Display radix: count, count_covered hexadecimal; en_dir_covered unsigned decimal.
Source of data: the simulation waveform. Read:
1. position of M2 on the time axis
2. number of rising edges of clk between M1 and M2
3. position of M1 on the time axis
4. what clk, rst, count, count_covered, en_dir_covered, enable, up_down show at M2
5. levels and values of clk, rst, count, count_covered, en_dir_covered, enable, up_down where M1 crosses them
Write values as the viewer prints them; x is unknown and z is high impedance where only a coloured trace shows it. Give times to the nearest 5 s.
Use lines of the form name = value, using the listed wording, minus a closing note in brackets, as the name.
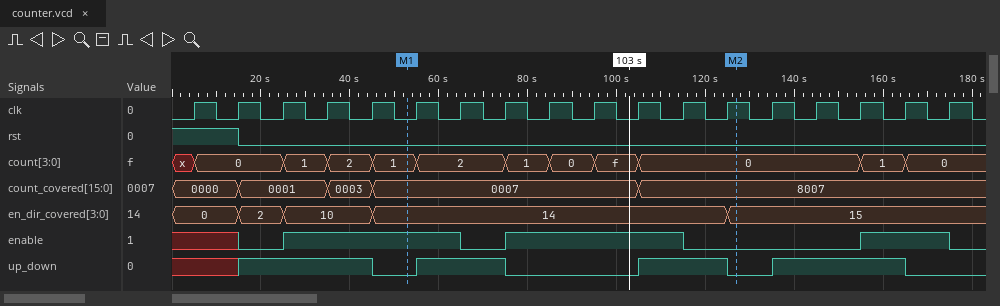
position of M2 on the time axis = 125 s
number of rising edges of clk between M1 and M2 = 8
position of M1 on the time axis = 55 s
what clk, rst, count, count_covered, en_dir_covered, enable, up_down show at M2 = clk=1, rst=0, count=0, count_covered=8007, en_dir_covered=15, enable=0, up_down=0
levels and values of clk, rst, count, count_covered, en_dir_covered, enable, up_down where M1 crosses them = clk=0, rst=0, count=1, count_covered=0007, en_dir_covered=14, enable=1, up_down=0
